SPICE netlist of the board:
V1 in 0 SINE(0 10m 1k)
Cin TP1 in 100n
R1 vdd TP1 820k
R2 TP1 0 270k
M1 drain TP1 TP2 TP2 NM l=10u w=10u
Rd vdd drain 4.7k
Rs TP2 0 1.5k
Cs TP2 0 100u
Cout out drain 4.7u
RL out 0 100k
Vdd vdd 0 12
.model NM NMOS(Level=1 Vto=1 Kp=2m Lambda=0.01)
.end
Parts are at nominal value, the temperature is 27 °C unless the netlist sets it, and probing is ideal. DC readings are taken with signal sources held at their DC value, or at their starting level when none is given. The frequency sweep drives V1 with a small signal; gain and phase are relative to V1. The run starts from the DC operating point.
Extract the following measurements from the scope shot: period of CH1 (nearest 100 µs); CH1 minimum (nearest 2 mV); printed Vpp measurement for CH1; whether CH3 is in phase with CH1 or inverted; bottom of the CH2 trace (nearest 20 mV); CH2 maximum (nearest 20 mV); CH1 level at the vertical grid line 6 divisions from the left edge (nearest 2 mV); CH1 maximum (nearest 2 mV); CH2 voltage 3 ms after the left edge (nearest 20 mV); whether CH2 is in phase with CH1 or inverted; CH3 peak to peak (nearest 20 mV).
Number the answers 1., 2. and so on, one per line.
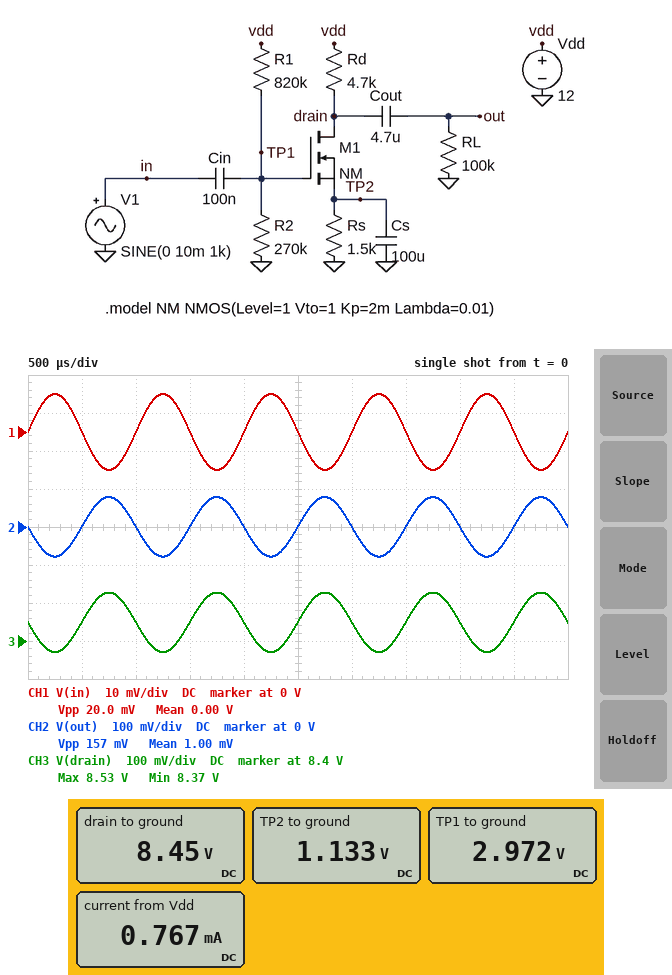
1. 1.0 ms
2. -10 mV
3. 20.0 mV
4. inverted
5. -80 mV
6. 80 mV
7. 0 V
8. 10 mV
9. 0 V
10. inverted
11. 160 mV
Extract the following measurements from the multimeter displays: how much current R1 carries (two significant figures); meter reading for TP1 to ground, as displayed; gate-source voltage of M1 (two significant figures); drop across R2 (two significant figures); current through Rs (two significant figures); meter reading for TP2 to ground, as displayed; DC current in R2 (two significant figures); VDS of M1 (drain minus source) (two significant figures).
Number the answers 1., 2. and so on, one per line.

1. 11 µA
2. 2.972 V
3. 1.8 V
4. 3.0 V
5. 760 µA
6. 1.133 V
7. 11 µA
8. 7.3 V
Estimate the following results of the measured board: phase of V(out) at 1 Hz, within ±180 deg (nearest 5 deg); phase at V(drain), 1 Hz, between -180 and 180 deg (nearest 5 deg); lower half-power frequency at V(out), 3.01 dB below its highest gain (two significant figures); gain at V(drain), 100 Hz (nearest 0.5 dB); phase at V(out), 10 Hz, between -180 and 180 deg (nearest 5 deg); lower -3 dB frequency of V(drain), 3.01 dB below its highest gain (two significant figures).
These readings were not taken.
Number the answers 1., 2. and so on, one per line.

1. -50 deg
2. -70 deg
3. 9.2 Hz
4. 18.0 dB
5. -125 deg
6. 9.2 Hz
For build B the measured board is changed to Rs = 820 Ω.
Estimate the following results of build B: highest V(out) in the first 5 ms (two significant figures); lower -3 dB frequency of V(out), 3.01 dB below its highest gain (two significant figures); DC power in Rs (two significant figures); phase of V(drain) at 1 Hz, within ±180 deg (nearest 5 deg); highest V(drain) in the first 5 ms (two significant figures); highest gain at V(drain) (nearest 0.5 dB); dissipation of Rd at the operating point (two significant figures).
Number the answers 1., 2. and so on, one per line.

1. 95 mV
2. 10 Hz
3. 1.1 mW
4. -80 deg
5. 6.7 V
6. 19.5 dB
7. 6.1 mW
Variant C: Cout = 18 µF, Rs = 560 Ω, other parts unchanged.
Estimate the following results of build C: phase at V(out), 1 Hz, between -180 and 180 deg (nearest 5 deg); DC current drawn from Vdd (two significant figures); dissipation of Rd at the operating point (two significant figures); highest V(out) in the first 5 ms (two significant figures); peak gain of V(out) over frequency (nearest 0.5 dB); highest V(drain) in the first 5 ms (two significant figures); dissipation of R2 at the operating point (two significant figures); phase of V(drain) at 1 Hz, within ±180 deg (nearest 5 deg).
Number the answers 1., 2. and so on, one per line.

1. -80 deg
2. 1.4 mA
3. 9.6 mW
4. 100 mV
5. 20.5 dB
6. 5.4 V
7. 33 µW
8. -85 deg
